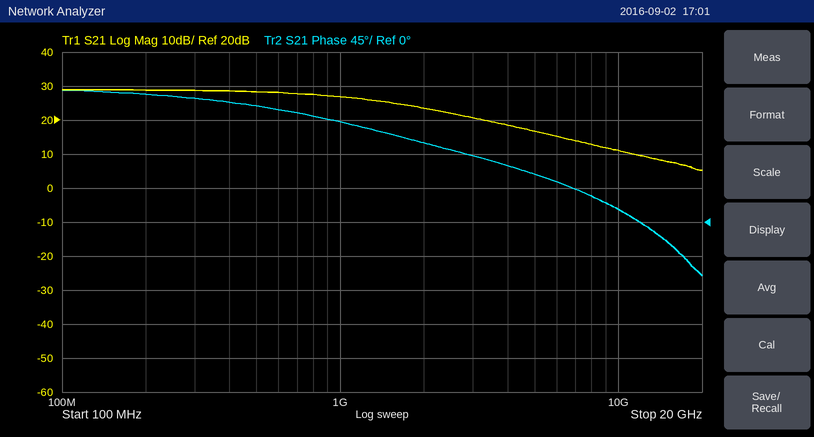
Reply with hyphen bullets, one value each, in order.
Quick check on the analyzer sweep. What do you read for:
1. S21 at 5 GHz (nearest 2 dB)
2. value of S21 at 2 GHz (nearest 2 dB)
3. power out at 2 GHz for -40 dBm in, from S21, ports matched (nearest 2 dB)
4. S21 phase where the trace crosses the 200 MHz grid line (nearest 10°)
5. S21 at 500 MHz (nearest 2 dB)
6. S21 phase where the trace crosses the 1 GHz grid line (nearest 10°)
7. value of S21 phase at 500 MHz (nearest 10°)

- 16 dB
- 24 dB
- -16 dBm
- 170°
- 28 dB
- 130°
- 150°
